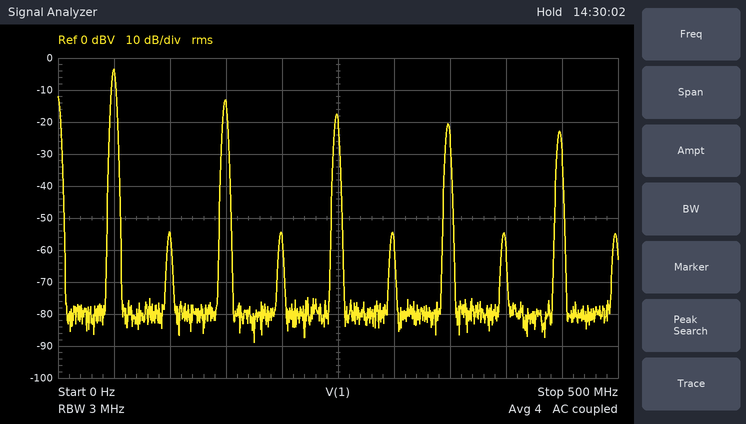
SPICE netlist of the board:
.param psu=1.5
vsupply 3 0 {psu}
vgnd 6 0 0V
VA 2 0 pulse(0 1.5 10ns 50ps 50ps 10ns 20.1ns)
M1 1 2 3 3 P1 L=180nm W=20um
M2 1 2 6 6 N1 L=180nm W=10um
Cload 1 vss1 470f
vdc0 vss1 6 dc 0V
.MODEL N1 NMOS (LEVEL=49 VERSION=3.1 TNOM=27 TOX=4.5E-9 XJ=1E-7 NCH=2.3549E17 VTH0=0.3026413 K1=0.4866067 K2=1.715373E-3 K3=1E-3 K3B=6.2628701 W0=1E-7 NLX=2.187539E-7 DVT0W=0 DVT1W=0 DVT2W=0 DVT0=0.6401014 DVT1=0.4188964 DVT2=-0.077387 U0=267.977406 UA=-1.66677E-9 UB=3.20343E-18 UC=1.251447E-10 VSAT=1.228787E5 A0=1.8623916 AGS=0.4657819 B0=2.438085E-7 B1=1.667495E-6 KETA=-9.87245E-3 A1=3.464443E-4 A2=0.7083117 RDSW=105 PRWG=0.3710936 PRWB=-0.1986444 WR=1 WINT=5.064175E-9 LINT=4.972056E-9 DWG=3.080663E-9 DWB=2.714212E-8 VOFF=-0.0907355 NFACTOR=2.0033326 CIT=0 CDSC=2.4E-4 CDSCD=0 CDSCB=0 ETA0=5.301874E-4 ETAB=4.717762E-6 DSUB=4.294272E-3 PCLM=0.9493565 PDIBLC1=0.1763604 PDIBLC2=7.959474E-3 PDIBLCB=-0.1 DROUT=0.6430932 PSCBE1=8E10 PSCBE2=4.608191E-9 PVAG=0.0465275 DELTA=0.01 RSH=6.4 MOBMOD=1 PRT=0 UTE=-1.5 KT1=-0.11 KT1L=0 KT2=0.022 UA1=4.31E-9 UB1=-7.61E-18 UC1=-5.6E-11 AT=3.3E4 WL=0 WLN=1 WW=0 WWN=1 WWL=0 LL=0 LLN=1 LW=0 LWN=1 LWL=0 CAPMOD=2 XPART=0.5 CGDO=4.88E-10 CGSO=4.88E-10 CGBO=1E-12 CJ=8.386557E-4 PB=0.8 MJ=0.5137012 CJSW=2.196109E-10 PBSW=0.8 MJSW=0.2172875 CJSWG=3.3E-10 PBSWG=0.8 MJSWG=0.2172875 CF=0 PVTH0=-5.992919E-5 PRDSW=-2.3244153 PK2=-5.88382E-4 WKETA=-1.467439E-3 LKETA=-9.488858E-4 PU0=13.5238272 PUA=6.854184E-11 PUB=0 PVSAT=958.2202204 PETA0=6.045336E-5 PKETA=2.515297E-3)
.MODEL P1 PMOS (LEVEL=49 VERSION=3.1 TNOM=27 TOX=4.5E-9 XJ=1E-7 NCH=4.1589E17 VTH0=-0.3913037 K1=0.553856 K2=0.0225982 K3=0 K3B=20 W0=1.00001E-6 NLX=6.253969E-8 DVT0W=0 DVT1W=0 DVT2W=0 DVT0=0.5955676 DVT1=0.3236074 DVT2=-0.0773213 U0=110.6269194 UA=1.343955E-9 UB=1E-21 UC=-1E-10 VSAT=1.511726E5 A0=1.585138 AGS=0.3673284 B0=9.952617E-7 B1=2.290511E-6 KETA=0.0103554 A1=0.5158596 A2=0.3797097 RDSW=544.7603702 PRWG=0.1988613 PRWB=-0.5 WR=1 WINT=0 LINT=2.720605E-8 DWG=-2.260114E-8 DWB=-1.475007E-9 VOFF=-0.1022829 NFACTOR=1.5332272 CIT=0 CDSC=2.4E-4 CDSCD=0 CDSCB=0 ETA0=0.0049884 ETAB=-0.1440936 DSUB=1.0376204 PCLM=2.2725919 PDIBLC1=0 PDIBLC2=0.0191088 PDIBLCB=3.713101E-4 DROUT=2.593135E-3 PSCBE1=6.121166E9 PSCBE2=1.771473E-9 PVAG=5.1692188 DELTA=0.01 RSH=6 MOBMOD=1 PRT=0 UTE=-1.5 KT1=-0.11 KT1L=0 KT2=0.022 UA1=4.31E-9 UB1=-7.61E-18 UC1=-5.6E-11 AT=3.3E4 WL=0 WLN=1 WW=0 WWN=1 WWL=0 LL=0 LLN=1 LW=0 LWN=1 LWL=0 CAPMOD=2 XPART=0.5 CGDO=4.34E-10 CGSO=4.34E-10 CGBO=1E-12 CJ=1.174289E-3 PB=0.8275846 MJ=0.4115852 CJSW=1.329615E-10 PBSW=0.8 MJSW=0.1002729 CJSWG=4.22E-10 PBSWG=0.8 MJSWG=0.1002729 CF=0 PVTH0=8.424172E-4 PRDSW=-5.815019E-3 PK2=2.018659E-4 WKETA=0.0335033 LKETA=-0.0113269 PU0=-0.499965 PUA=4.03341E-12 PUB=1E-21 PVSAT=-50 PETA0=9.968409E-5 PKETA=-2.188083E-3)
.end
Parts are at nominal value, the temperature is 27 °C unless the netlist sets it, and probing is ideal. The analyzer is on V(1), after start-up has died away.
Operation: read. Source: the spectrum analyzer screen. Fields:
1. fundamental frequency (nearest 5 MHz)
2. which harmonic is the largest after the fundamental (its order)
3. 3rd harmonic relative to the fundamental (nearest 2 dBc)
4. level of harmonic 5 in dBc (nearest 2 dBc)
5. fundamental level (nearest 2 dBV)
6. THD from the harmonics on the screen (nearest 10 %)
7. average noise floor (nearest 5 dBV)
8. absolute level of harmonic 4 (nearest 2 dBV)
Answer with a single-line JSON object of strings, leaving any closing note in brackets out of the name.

{"fundamental frequency": "50 MHz", "which harmonic is the largest after the fundamental": "3", "3rd harmonic relative to the fundamental": "-10 dBc", "level of harmonic 5 in dBc": "-14 dBc", "fundamental level": "-4 dBV", "THD from the harmonics on the screen": "40 %", "average noise floor": "-80 dBV", "absolute level of harmonic 4": "-54 dBV"}
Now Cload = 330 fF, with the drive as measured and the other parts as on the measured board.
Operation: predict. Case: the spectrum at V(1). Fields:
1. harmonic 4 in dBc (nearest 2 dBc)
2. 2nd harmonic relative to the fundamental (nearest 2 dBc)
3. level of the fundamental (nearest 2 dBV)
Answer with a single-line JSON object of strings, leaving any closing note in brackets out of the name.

{"harmonic 4 in dBc": "-54 dBc", "2nd harmonic relative to the fundamental": "-54 dBc", "level of the fundamental": "-4 dBV"}
